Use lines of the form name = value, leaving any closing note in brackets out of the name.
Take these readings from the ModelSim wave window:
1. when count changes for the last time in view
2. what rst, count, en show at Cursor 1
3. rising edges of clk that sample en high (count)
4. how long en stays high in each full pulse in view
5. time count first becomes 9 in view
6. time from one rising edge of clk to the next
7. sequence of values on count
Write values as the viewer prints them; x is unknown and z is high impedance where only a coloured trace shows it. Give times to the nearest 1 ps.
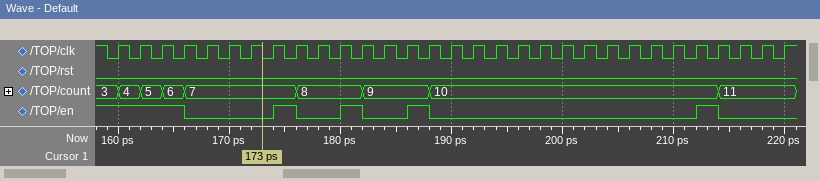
when count changes for the last time in view = 214 ps
what rst, count, en show at Cursor 1 = rst=0, count=7, en=0
rising edges of clk that sample en high = 8
how long en stays high in each full pulse in view = 2 ps, 2 ps, 2 ps, 2 ps
time count first becomes 9 in view = 182 ps
time from one rising edge of clk to the next = 2 ps
sequence of values on count = 3, 4, 5, 6, 7, 8, 9, 10, 11
